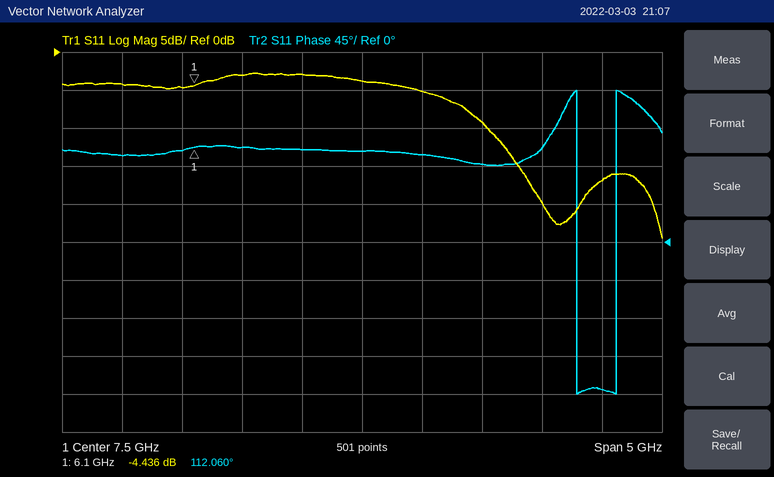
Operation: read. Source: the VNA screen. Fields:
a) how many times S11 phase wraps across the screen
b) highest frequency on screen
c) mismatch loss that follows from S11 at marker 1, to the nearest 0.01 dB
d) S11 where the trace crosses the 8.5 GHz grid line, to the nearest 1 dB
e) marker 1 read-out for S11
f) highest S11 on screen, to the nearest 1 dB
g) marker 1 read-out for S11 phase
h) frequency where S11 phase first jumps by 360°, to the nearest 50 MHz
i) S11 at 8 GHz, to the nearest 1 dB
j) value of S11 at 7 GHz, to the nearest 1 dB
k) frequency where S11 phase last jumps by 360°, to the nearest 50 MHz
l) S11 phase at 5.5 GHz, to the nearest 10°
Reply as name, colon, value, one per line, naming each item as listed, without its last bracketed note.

how many times S11 phase wraps across the screen: 2
highest frequency on screen: 10 GHz
mismatch loss that follows from S11 at marker 1, to the nearest 0.01 dB: 1.94 dB
S11 where the trace crosses the 8.5 GHz grid line, to the nearest 1 dB: -9 dB
marker 1 read-out for S11: -4.436 dB
highest S11 on screen, to the nearest 1 dB: -3 dB
marker 1 read-out for S11 phase: 112.060°
frequency where S11 phase first jumps by 360°, to the nearest 50 MHz: 9.30 GHz
S11 at 8 GHz, to the nearest 1 dB: -5 dB
value of S11 at 7 GHz, to the nearest 1 dB: -3 dB
frequency where S11 phase last jumps by 360°, to the nearest 50 MHz: 9.60 GHz
S11 phase at 5.5 GHz, to the nearest 10°: 100°
